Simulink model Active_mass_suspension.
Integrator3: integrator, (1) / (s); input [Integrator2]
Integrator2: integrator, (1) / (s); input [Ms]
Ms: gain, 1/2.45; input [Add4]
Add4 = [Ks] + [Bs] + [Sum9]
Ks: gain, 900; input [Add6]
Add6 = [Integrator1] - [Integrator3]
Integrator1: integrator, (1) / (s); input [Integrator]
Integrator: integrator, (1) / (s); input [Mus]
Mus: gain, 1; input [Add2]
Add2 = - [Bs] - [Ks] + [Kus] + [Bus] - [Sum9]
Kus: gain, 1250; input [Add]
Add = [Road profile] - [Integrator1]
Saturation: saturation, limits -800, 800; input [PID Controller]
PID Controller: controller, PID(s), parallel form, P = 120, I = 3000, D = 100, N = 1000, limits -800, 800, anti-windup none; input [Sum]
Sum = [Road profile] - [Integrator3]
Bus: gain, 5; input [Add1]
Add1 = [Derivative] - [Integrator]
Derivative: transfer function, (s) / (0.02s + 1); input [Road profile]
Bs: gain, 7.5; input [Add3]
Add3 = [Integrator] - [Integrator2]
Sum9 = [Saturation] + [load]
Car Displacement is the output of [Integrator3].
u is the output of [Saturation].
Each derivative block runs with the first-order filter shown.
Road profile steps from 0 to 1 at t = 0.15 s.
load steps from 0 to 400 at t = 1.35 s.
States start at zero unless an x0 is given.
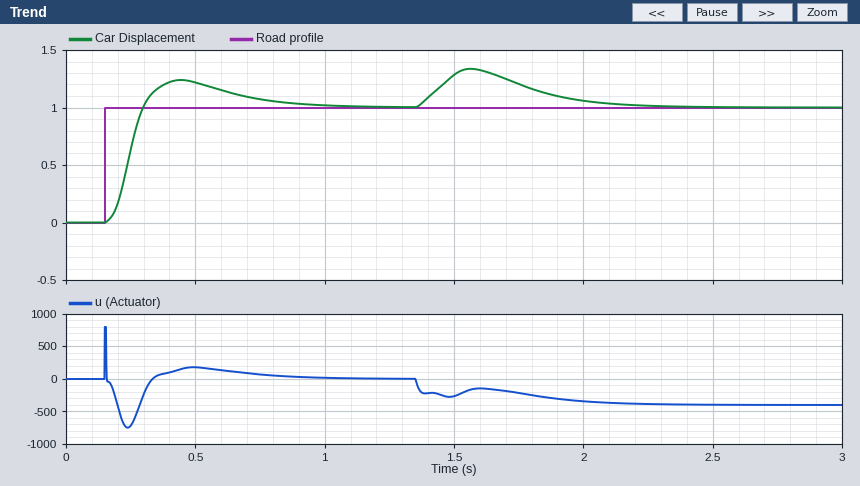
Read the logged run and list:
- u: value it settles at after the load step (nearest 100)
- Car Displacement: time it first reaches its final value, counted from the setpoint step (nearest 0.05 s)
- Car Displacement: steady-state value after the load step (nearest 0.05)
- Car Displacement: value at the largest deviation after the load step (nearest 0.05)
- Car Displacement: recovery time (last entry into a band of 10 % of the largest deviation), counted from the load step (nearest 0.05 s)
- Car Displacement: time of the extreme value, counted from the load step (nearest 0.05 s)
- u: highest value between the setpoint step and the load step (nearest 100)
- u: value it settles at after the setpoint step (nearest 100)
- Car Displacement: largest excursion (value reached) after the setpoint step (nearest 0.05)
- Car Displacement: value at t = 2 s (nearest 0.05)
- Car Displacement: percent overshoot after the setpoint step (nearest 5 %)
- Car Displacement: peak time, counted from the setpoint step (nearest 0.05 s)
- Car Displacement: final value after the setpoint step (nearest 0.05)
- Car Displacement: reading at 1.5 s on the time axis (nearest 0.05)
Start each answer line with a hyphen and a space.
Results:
- -400
- 0.15 s
- 1.00
- 1.35
- 0.75 s
- 0.20 s
- 800
- 0
- 1.25
- 1.05
- 25 %
- 0.30 s
- 1.00
- 1.30
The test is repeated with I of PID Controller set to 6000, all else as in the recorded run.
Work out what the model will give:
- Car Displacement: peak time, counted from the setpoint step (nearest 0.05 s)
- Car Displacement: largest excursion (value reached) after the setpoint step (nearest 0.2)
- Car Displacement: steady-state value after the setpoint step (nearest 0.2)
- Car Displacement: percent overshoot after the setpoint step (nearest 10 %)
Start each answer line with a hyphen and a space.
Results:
- 0.25 s
- 1.4
- 1.0
- 40 %
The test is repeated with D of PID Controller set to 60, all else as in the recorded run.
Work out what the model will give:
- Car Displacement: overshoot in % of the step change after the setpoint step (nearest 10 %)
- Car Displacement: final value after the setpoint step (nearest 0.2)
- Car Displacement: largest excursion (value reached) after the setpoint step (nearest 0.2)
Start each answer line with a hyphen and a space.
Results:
- 40 %
- 1.0
- 1.4
